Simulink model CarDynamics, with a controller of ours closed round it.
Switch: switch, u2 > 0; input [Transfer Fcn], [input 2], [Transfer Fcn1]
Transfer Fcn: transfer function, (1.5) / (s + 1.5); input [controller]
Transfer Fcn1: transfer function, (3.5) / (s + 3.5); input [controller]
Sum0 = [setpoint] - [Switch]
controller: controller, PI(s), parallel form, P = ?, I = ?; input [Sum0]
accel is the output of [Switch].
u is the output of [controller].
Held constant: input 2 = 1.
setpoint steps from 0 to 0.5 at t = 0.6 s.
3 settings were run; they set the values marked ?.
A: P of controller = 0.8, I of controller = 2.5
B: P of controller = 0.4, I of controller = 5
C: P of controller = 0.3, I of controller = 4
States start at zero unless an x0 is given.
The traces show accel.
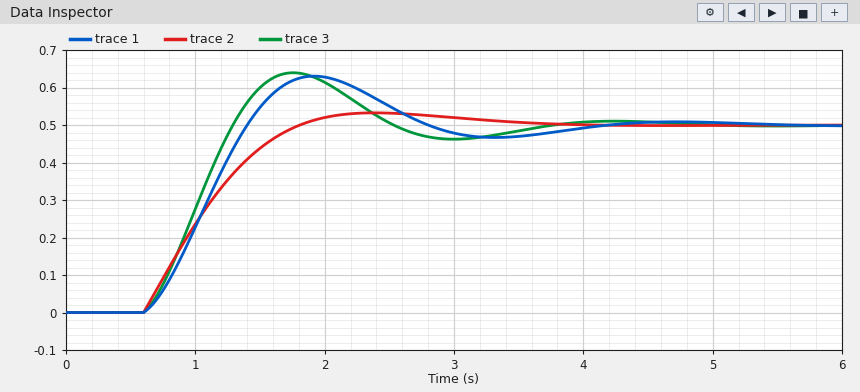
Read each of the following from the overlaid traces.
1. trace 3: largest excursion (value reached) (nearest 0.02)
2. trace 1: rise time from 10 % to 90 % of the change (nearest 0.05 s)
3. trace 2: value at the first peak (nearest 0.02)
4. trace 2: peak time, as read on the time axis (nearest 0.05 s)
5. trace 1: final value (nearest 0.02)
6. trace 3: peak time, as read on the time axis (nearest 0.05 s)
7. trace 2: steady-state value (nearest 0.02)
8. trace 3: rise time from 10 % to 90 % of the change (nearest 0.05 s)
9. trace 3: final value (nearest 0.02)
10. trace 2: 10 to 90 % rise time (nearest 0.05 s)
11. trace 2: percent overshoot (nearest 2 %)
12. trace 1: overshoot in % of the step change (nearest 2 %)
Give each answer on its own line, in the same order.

0.64
0.60 s
0.54
2.40 s
0.50
1.75 s
0.50
0.50 s
0.50
0.85 s
6 %
26 %
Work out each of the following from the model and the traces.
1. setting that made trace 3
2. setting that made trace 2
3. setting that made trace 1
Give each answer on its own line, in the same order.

B
A
C
